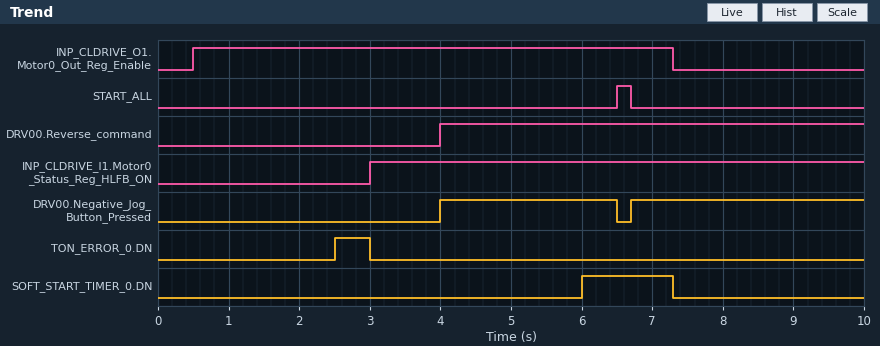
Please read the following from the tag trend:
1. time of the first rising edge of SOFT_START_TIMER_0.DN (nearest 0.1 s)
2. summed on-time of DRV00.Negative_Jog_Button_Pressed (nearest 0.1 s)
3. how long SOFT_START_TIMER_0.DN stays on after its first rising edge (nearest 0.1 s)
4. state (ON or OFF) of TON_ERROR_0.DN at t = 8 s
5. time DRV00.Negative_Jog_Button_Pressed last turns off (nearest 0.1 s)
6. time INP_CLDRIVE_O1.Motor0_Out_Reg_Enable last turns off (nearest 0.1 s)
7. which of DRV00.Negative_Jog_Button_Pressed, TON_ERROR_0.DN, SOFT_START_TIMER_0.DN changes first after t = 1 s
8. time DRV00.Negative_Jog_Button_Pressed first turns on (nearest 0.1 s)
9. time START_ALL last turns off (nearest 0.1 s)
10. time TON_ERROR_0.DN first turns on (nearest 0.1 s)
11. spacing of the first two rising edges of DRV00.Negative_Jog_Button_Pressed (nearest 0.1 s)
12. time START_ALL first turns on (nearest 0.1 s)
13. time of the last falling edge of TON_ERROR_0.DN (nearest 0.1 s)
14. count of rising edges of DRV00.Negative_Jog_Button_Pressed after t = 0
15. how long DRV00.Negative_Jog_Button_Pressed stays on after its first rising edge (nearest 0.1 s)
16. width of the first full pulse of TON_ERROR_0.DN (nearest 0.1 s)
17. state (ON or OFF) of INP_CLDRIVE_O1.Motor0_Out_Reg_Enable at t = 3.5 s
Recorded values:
6.0 s
5.8 s
1.3 s
OFF
6.5 s
7.3 s
TON_ERROR_0.DN
4.0 s
6.7 s
2.5 s
2.7 s
6.5 s
3.0 s
2
2.5 s
0.5 s
ON
